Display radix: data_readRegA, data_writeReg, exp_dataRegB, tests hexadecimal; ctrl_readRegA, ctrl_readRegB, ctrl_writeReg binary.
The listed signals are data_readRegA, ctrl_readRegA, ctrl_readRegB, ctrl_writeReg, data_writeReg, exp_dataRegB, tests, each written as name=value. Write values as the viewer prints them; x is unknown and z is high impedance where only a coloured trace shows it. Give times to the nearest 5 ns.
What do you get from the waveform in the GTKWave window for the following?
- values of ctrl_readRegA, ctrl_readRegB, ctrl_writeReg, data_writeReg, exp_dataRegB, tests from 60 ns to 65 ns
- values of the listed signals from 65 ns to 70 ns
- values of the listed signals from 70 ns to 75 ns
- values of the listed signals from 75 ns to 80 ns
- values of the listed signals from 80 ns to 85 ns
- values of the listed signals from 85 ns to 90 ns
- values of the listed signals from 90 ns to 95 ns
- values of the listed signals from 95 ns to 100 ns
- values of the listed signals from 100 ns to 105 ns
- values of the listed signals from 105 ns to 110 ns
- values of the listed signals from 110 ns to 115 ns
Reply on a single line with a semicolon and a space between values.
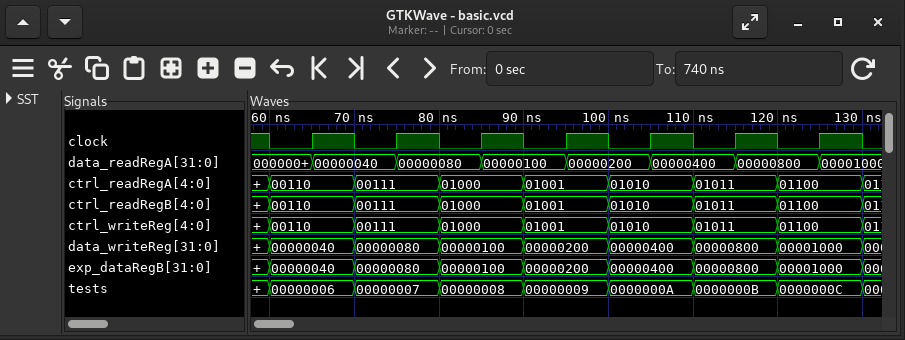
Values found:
ctrl_readRegA=00110, ctrl_readRegB=00110, ctrl_writeReg=00110, data_writeReg=00000040, exp_dataRegB=00000040, tests=00000006; data_readRegA=00000040, ctrl_readRegA=00110, ctrl_readRegB=00110, ctrl_writeReg=00110, data_writeReg=00000040, exp_dataRegB=00000040, tests=00000006; data_readRegA=00000040, ctrl_readRegA=00111, ctrl_readRegB=00111, ctrl_writeReg=00111, data_writeReg=00000080, exp_dataRegB=00000080, tests=00000007; data_readRegA=00000080, ctrl_readRegA=00111, ctrl_readRegB=00111, ctrl_writeReg=00111, data_writeReg=00000080, exp_dataRegB=00000080, tests=00000007; data_readRegA=00000080, ctrl_readRegA=01000, ctrl_readRegB=01000, ctrl_writeReg=01000, data_writeReg=00000100, exp_dataRegB=00000100, tests=00000008; data_readRegA=00000100, ctrl_readRegA=01000, ctrl_readRegB=01000, ctrl_writeReg=01000, data_writeReg=00000100, exp_dataRegB=00000100, tests=00000008; data_readRegA=00000100, ctrl_readRegA=01001, ctrl_readRegB=01001, ctrl_writeReg=01001, data_writeReg=00000200, exp_dataRegB=00000200, tests=00000009; data_readRegA=00000200, ctrl_readRegA=01001, ctrl_readRegB=01001, ctrl_writeReg=01001, data_writeReg=00000200, exp_dataRegB=00000200, tests=00000009; data_readRegA=00000200, ctrl_readRegA=01010, ctrl_readRegB=01010, ctrl_writeReg=01010, data_writeReg=00000400, exp_dataRegB=00000400, tests=0000000A; data_readRegA=00000400, ctrl_readRegA=01010, ctrl_readRegB=01010, ctrl_writeReg=01010, data_writeReg=00000400, exp_dataRegB=00000400, tests=0000000A; data_readRegA=00000400, ctrl_readRegA=01011, ctrl_readRegB=01011, ctrl_writeReg=01011, data_writeReg=00000800, exp_dataRegB=00000800, tests=0000000B
